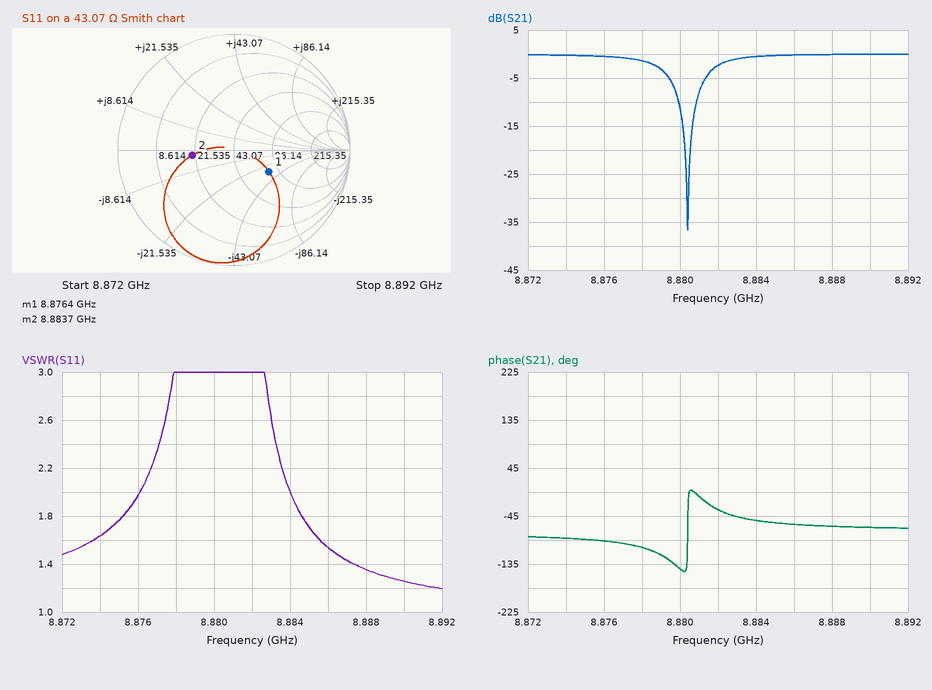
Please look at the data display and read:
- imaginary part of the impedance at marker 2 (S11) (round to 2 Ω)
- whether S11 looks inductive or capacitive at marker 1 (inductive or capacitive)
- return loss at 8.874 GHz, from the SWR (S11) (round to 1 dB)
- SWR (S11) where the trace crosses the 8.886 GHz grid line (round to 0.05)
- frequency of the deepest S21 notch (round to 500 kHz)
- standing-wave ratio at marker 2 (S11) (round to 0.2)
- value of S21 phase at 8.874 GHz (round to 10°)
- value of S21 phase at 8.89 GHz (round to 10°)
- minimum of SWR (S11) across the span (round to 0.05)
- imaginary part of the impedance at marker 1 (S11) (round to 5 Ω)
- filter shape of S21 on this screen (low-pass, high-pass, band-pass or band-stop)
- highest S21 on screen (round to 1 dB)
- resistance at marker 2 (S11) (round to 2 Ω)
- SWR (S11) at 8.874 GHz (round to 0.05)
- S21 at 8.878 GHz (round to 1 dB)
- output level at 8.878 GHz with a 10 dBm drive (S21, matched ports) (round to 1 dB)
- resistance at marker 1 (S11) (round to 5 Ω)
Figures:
-2 Ω
capacitive
12 dB
1.55
8.8805 GHz
2.2
-90°
-70°
1.20
-30 Ω
band-stop
0 dB
20 Ω
1.65
-1 dB
9 dBm
70 Ω
